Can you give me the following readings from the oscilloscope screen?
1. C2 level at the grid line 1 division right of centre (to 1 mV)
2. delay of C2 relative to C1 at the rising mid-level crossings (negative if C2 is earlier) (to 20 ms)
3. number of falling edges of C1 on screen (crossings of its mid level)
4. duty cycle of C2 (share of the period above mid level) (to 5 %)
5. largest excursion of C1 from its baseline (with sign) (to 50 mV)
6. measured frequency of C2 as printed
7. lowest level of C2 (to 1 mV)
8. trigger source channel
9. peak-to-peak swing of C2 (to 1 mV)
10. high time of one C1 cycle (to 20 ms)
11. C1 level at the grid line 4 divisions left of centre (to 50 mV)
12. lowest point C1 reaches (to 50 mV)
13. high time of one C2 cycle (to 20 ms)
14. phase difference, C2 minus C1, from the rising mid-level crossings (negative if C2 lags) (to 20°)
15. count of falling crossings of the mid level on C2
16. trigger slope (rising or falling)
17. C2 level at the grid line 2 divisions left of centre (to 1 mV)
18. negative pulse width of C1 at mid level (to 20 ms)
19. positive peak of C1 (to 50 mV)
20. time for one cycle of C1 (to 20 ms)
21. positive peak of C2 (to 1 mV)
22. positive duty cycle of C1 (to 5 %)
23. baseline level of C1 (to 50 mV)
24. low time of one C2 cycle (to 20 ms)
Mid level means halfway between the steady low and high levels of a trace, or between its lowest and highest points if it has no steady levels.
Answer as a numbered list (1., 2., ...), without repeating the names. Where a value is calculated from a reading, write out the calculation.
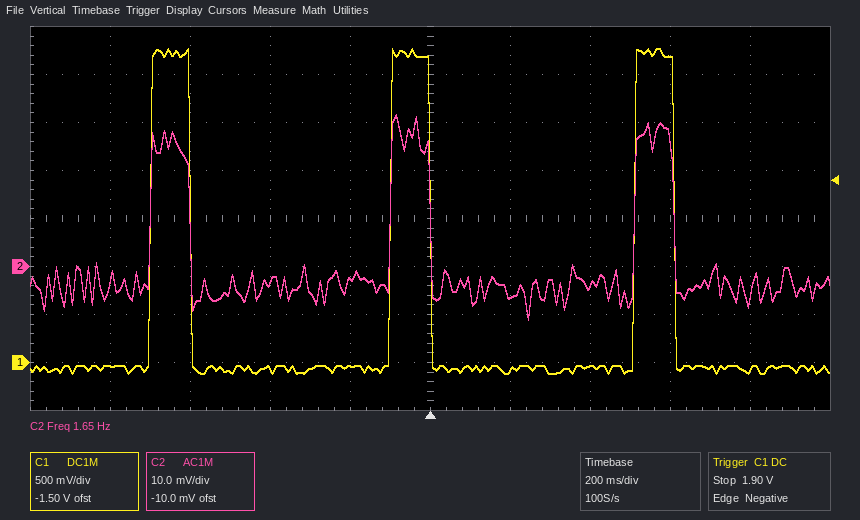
1. -6 mV
2. 0 ms
3. 3
4. 15 %
5. 3.25 V − (-50 mV) = +3.30 V
6. 1.65 Hz
7. -11 mV
8. C1
9. 32 mV − (-11 mV) = 43 mV
10. 100 ms
11. -50 mV
12. -100 mV
13. 100 ms
14. −360° × (0 ms) / 600 ms ≈ 0°
15. 3
16. falling
17. -3 mV
18. 500 ms
19. 3.25 V
20. 600 ms
21. 32 mV
22. 100 ms / 600 ms ≈ 16.7 %, so 15 % to the nearest 5 %
23. -50 mV
24. 500 ms
